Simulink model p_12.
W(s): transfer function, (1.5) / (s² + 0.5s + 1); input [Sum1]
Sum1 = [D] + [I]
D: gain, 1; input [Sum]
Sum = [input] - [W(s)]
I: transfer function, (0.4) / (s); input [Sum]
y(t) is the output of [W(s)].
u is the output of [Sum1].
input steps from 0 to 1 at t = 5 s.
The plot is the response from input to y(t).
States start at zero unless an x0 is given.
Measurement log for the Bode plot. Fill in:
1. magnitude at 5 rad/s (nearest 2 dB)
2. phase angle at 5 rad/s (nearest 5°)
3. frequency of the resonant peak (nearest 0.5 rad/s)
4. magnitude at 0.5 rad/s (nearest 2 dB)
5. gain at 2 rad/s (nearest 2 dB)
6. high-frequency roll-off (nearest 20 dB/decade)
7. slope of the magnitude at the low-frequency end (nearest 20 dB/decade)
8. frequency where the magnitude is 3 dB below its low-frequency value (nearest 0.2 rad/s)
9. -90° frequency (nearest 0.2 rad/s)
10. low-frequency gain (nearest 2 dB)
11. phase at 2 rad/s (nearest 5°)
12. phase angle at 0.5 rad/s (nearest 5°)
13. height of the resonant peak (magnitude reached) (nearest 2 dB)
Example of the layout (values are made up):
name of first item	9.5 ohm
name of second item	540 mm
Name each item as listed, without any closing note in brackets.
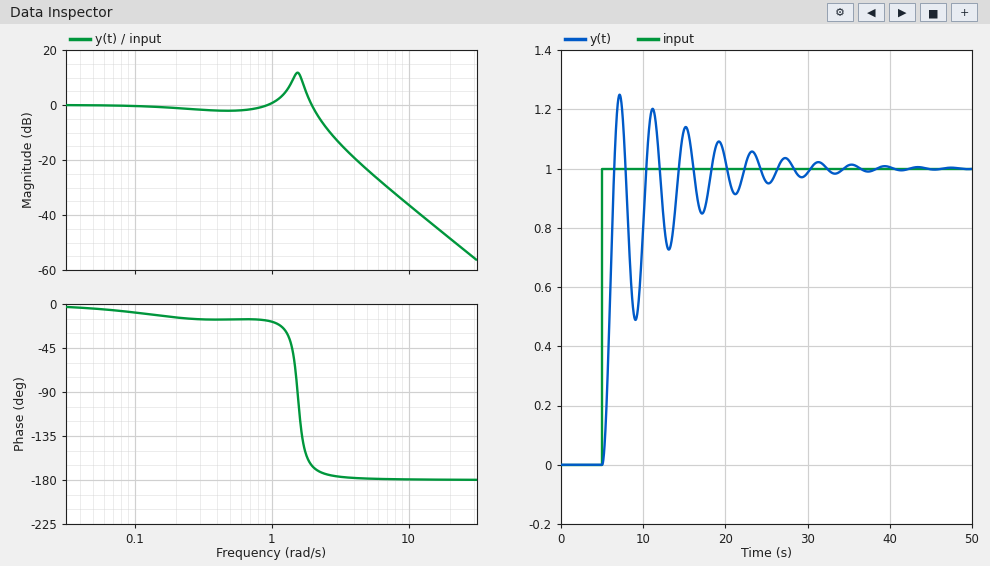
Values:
magnitude at 5 rad/s	-24 dB
phase angle at 5 rad/s	-180°
frequency of the resonant peak	1.5 rad/s
magnitude at 0.5 rad/s	-2 dB
gain at 2 rad/s	0 dB
high-frequency roll-off	-40 dB/decade
slope of the magnitude at the low-frequency end	0 dB/decade
frequency where the magnitude is 3 dB below its low-frequency value	2.2 rad/s
-90° frequency	1.6 rad/s
low-frequency gain	0 dB
phase at 2 rad/s	-165°
phase angle at 0.5 rad/s	-15°
height of the resonant peak (magnitude reached)	12 dB
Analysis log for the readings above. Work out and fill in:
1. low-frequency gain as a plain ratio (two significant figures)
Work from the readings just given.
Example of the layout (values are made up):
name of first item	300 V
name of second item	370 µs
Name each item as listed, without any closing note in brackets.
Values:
low-frequency gain as a plain ratio	1.0
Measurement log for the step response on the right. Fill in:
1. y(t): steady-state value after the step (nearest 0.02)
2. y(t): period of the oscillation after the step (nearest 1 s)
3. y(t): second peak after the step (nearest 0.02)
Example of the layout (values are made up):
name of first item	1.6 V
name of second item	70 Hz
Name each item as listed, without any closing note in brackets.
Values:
y(t): steady-state value after the step	1.00
y(t): period of the oscillation after the step	4 s
y(t): second peak after the step	1.20
